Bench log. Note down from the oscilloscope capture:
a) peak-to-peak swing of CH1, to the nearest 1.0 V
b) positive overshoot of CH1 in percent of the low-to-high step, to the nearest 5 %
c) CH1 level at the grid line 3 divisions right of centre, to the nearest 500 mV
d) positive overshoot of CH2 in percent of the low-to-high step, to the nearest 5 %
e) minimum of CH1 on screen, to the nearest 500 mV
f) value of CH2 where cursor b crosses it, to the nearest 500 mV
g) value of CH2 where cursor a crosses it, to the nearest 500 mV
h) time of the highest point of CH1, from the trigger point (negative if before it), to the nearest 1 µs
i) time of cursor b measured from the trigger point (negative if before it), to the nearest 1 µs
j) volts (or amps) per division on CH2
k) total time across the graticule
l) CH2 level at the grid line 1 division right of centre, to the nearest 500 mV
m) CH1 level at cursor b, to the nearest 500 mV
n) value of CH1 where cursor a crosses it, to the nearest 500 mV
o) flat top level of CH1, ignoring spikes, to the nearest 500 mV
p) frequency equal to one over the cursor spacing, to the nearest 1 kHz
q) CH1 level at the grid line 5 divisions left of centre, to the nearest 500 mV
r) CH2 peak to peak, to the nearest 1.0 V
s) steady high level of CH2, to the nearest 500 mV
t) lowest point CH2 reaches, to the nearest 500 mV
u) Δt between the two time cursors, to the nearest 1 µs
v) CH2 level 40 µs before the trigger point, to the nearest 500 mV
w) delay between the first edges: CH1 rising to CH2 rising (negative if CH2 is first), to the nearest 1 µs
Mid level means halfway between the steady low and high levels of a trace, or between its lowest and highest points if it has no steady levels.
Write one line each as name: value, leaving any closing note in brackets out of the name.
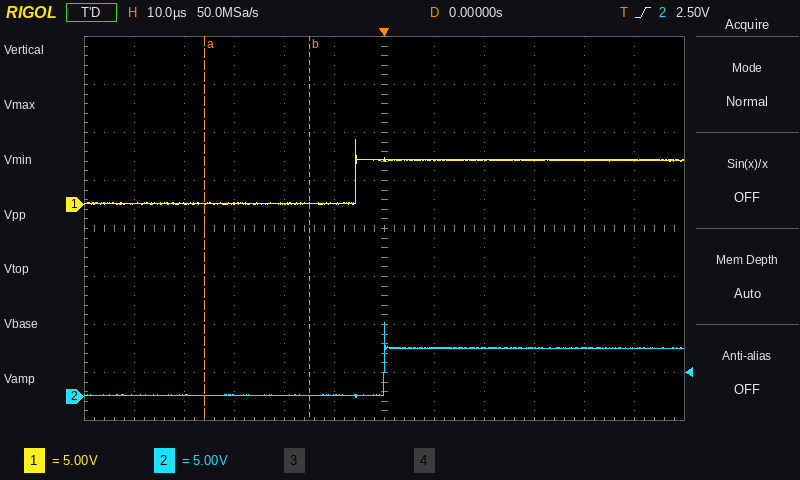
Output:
peak-to-peak swing of CH1, to the nearest 1.0 V: 7.0 V
positive overshoot of CH1 in percent of the low-to-high step, to the nearest 5 %: 45 %
CH1 level at the grid line 3 divisions right of centre, to the nearest 500 mV: 4.5 V
positive overshoot of CH2 in percent of the low-to-high step, to the nearest 5 %: 55 %
minimum of CH1 on screen, to the nearest 500 mV: 0.0 V
value of CH2 where cursor b crosses it, to the nearest 500 mV: 0.0 V
value of CH2 where cursor a crosses it, to the nearest 500 mV: 0.0 V
time of the highest point of CH1, from the trigger point (negative if before it), to the nearest 1 µs: -6 µs
time of cursor b measured from the trigger point (negative if before it), to the nearest 1 µs: -15 µs
volts (or amps) per division on CH2: 5 V
total time across the graticule: 120 µs
CH2 level at the grid line 1 division right of centre, to the nearest 500 mV: 5.0 V
CH1 level at cursor b, to the nearest 500 mV: 0.0 V
value of CH1 where cursor a crosses it, to the nearest 500 mV: 0.0 V
flat top level of CH1, ignoring spikes, to the nearest 500 mV: 4.5 V
frequency equal to one over the cursor spacing, to the nearest 1 kHz: 48 kHz
CH1 level at the grid line 5 divisions left of centre, to the nearest 500 mV: 0.0 V
CH2 peak to peak, to the nearest 1.0 V: 8.0 V
steady high level of CH2, to the nearest 500 mV: 5.0 V
lowest point CH2 reaches, to the nearest 500 mV: 0.0 V
Δt between the two time cursors, to the nearest 1 µs: 21 µs
CH2 level 40 µs before the trigger point, to the nearest 500 mV: 0.0 V
delay between the first edges: CH1 rising to CH2 rising (negative if CH2 is first), to the nearest 1 µs: +6 µs
